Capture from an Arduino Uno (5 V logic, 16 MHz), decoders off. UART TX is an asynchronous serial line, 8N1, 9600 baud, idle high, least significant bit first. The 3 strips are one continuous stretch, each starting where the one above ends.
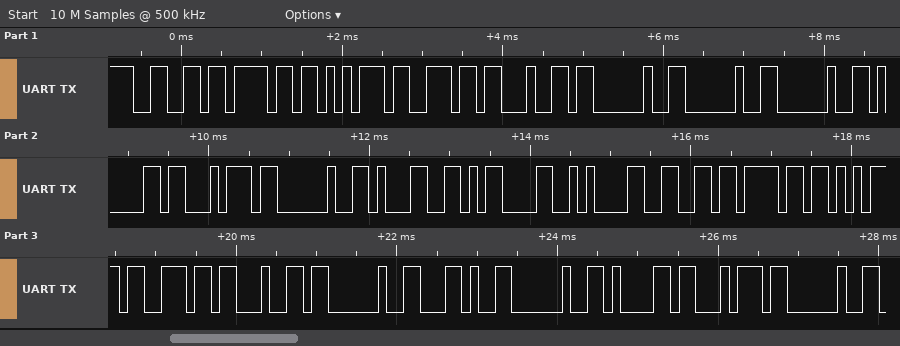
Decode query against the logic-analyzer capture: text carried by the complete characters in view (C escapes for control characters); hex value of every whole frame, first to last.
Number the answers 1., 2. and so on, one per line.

1. "found   at 1\r\nfound , at "
2. 66 6F 75 6E 64 20 20 20 61 74 20 31 0D 0A 66 6F 75 6E 64 20 2C 20 61 74 20
